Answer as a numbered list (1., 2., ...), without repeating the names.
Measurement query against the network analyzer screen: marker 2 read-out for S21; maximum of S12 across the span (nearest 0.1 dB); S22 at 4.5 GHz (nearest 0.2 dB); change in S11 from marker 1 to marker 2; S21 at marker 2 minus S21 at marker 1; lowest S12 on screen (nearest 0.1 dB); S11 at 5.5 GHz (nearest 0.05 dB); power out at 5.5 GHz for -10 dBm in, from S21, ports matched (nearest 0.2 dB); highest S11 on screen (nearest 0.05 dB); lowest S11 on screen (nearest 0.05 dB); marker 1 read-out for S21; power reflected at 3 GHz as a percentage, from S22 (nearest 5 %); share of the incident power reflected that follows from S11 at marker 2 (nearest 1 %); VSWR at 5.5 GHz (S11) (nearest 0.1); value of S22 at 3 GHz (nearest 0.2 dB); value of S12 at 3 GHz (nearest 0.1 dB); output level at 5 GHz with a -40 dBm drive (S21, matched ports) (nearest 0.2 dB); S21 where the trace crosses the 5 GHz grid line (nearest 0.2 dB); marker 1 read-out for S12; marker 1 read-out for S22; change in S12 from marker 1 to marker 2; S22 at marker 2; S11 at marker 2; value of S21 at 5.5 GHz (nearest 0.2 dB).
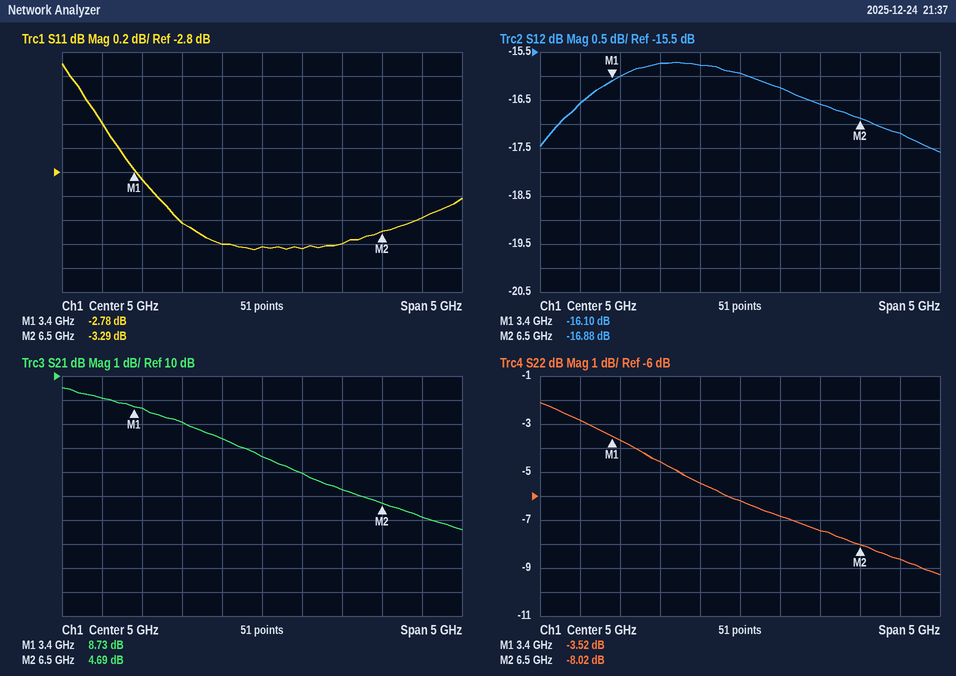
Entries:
1. 4.69 dB
2. -15.7 dB
3. -5.4 dB
4. -0.51 dB
5. -4.04 dB
6. -17.6 dB
7. -3.45 dB
8. -4.0 dBm
9. -1.90 dB
10. -3.45 dB
11. 8.73 dB
12. 50 %
13. 47 %
14. 5.1
15. -2.8 dB
16. -16.6 dB
17. -33.4 dBm
18. 6.6 dB
19. -16.10 dB
20. -3.52 dB
21. -0.78 dB
22. -8.02 dB
23. -3.29 dB
24. 6.0 dB
